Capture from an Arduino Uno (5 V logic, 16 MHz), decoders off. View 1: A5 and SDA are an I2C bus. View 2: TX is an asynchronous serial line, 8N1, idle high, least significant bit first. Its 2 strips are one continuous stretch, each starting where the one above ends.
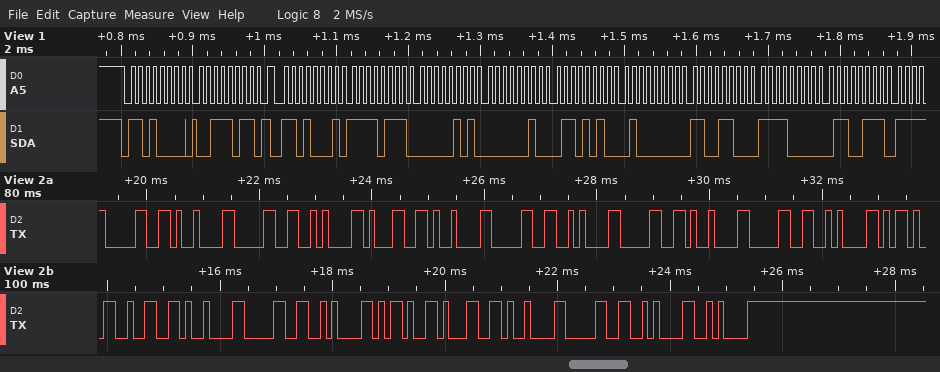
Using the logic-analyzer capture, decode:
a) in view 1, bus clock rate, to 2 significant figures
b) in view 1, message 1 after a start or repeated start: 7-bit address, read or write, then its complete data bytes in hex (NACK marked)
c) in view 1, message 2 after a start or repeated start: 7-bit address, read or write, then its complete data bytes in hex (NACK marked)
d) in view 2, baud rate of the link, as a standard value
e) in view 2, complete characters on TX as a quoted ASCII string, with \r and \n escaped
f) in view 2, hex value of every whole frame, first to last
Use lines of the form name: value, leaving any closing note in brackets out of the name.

in view 1, bus clock rate, to 2 significant figures: 100 kHz
in view 1, message 1 after a start or repeated start: 7-bit address, read or write, then its complete data bytes in hex: 0x68 write: 3B
in view 1, message 2 after a start or repeated start: 7-bit address, read or write, then its complete data bytes in hex: 0x68 read: F7 05 02 6A 40 CC F0 67
in view 2, baud rate of the link, as a standard value: 9600 baud
in view 2, complete characters on TX as a quoted ASCII string, with \r and \n escaped: "0\t0\n1\t0\n0\t0\n-2\t0\n-1\t0\n\n"
in view 2, hex value of every whole frame, first to last: 30 09 30 0A 31 09 30 0A 30 09 30 0A 2D 32 09 30 0A 2D 31 09 30 0A 0A
